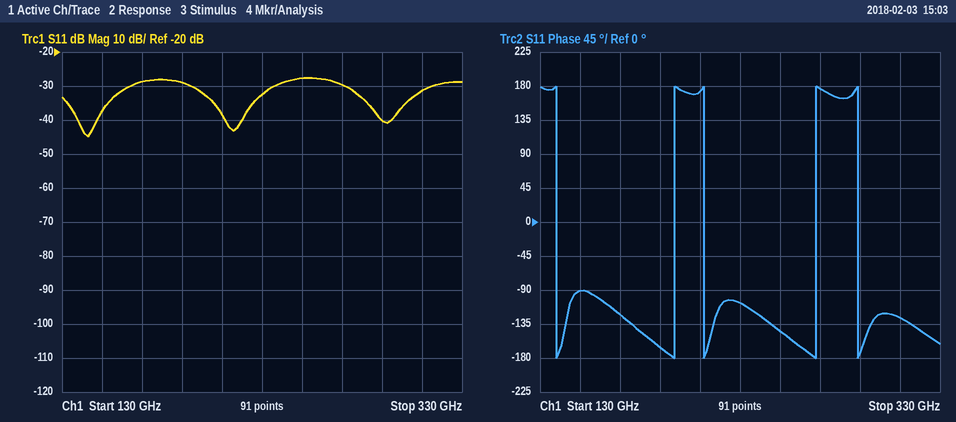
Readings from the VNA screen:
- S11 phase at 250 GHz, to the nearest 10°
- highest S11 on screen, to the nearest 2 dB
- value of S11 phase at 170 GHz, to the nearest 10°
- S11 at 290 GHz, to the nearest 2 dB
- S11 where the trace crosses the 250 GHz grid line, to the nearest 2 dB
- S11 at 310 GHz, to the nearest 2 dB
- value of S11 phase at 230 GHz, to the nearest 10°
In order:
-140°
-28 dB
-120°
-40 dB
-28 dB
-32 dB
-110°
